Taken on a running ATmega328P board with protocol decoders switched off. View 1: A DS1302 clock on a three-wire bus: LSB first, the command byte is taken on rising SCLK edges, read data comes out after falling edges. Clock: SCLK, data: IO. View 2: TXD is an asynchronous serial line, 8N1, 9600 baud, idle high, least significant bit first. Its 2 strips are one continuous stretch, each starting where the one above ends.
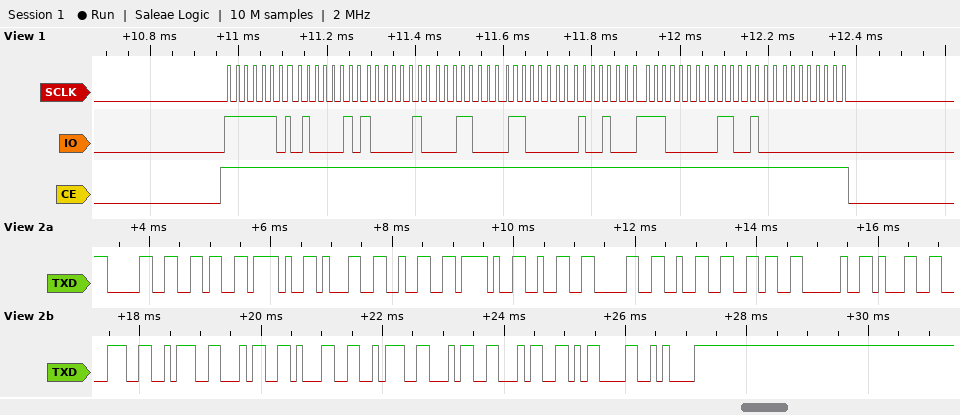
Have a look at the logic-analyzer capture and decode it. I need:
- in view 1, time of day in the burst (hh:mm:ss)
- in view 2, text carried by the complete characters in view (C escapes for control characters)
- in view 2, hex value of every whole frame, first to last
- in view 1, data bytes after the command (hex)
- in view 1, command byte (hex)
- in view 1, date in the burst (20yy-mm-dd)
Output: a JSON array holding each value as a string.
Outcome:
["18:41:42", "\"06/12/2026 18:41:44\\r\\n\"", "30 36 2F 31 32 2F 32 30 32 36 20 31 38 3A 34 31 3A 34 34 0D 0A", "42 41 18 06 12 07 26 00", "0xBF", "2026-12-06"]
